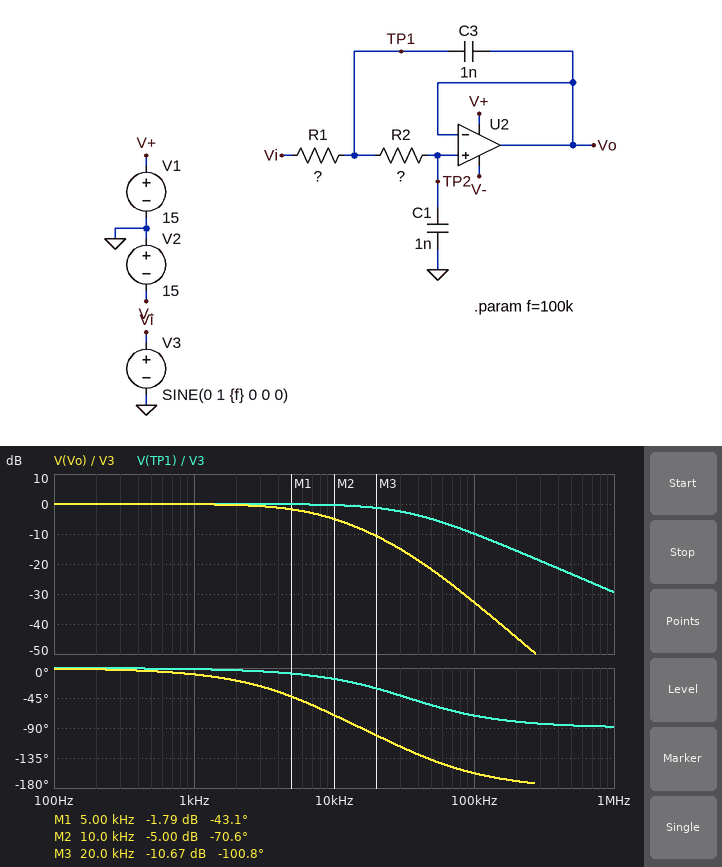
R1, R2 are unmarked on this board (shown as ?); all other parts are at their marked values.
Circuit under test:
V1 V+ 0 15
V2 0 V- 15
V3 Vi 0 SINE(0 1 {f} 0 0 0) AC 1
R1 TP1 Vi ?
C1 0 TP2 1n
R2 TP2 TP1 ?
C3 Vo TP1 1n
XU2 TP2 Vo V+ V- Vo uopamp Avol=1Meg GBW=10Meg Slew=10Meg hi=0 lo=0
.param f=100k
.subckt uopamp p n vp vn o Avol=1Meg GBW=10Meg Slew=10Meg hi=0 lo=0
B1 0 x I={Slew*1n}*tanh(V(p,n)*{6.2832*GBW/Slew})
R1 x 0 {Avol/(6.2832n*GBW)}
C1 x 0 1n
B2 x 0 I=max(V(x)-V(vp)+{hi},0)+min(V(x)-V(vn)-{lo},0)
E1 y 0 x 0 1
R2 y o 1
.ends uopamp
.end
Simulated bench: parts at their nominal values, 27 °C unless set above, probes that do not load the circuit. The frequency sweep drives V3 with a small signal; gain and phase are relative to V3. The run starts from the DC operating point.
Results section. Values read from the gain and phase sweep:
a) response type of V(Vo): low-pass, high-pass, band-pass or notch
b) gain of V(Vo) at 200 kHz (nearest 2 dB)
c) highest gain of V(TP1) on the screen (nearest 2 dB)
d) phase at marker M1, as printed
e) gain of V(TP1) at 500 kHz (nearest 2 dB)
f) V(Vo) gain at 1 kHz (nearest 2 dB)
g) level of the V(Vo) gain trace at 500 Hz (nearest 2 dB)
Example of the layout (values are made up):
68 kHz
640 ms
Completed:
low-pass
-44 dB
0 dB
-43.1 deg
-24 dB
0 dB
0 dB
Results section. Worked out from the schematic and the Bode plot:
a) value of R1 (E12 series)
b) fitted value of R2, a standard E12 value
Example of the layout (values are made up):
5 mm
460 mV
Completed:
4.7 kΩ
22 kΩ
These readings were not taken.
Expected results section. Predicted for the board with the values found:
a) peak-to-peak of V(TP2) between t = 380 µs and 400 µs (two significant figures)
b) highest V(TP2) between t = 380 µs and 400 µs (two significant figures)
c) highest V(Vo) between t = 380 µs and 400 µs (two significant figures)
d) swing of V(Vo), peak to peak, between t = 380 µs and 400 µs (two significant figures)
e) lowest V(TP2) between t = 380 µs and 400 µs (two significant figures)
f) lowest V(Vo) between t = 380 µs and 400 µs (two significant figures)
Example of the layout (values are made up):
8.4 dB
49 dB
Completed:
46 mV
23 mV
23 mV
46 mV
-23 mV
-23 mV
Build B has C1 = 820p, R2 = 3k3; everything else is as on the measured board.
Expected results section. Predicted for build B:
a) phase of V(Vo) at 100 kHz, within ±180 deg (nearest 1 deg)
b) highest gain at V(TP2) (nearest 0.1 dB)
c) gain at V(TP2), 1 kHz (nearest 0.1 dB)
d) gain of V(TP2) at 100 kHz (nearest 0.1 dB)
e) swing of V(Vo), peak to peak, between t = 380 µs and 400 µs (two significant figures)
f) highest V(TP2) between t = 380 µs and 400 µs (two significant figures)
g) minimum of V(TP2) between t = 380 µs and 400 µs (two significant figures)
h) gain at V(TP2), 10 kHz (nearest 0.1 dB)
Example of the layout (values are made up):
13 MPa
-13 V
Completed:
-135 deg
0 dB
0 dB
-15.2 dB
350 mV
170 mV
-170 mV
-0.3 dB
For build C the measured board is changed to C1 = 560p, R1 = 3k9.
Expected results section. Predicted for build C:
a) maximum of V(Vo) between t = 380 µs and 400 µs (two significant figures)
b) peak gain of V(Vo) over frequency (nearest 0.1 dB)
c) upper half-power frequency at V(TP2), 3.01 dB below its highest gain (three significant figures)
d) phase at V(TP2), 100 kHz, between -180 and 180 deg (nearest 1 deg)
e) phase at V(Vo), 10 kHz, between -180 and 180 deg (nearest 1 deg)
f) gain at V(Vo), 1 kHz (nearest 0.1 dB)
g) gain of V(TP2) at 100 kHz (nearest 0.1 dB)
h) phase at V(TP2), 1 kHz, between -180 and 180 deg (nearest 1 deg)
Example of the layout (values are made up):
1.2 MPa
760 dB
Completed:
50 mV
0 dB
13.9 kHz
-153 deg
-48 deg
0 dB
-26.1 dB
-5 deg
